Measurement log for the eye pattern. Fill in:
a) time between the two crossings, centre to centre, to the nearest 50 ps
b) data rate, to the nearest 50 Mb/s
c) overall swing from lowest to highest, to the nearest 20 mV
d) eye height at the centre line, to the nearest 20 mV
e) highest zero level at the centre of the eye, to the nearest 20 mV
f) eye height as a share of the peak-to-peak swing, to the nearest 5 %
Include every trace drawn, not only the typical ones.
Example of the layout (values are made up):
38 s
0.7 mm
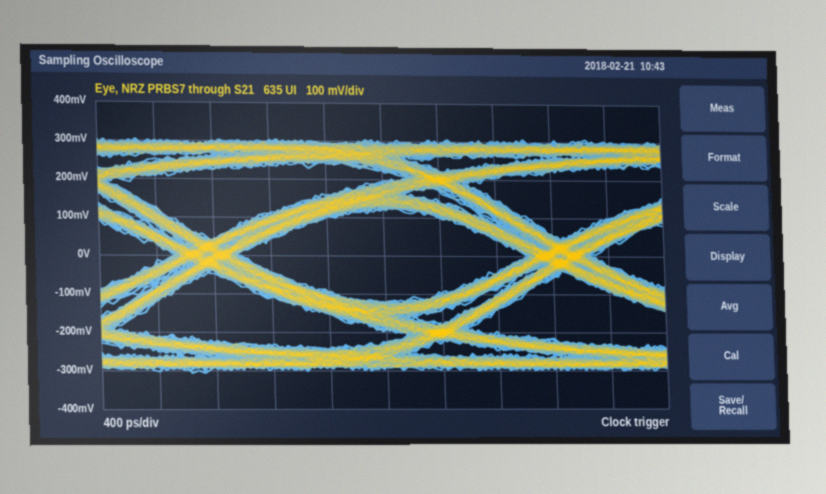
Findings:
2.50 ns
400 Mb/s
620 mV
240 mV
-120 mV
40 %
